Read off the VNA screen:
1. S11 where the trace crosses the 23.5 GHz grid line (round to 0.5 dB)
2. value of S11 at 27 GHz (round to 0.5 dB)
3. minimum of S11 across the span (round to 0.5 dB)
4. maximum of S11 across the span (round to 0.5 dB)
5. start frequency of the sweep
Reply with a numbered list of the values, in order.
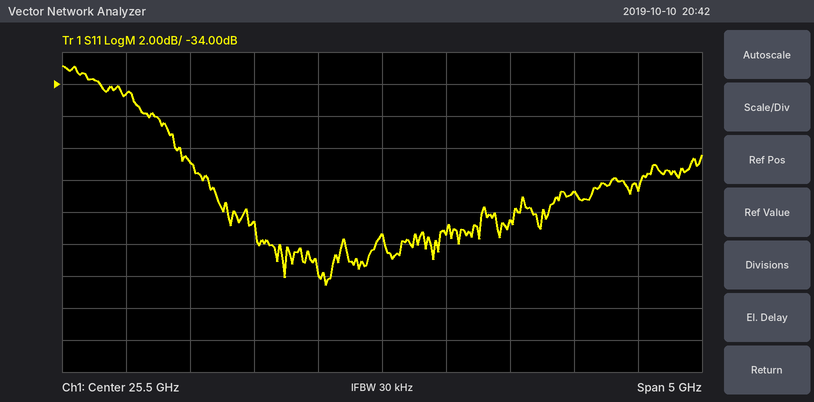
1. -34.5 dB
2. -40.5 dB
3. -46.5 dB
4. -33.0 dB
5. 23 GHz
